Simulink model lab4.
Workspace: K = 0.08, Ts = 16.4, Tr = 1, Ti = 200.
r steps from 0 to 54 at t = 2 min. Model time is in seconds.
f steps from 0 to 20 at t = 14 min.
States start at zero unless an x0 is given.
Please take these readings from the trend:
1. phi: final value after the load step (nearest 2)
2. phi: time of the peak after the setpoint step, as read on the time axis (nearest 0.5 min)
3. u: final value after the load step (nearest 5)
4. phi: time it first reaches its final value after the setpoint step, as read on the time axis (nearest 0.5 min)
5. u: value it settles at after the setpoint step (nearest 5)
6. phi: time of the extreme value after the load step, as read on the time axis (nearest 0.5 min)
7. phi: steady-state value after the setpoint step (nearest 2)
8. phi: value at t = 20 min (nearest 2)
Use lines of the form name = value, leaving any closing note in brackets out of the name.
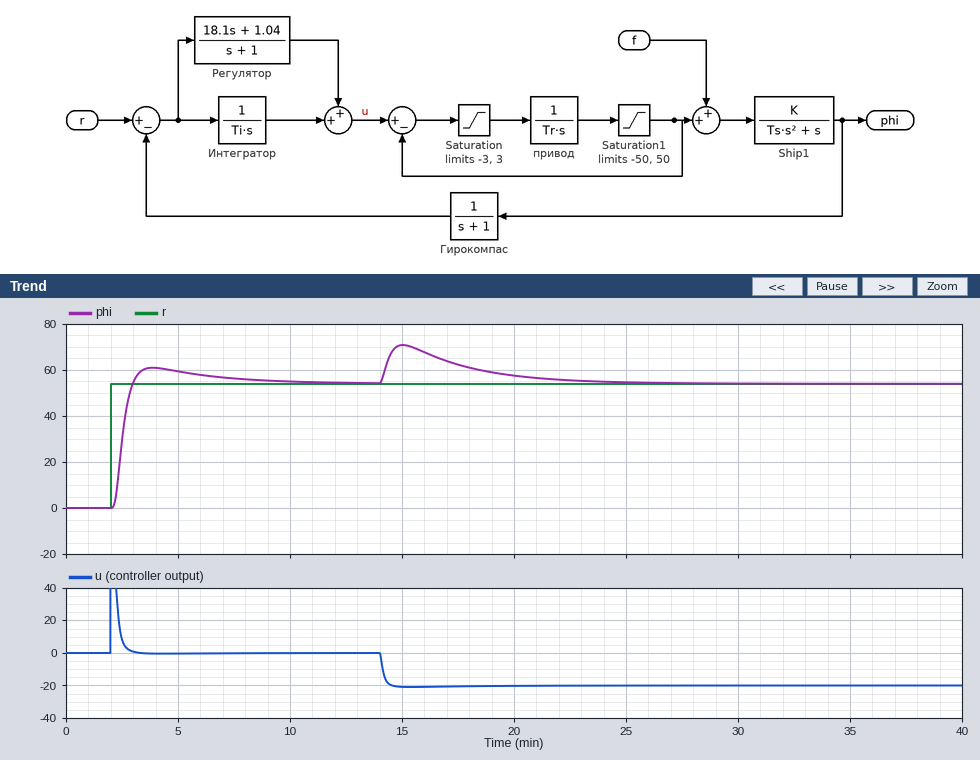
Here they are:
phi: final value after the load step = 54
phi: time of the peak after the setpoint step, as read on the time axis = 4.0 min
u: final value after the load step = -20
phi: time it first reaches its final value after the setpoint step, as read on the time axis = 3.0 min
u: value it settles at after the setpoint step = 0
phi: time of the extreme value after the load step, as read on the time axis = 15.0 min
phi: steady-state value after the setpoint step = 54
phi: value at t = 20 min = 58
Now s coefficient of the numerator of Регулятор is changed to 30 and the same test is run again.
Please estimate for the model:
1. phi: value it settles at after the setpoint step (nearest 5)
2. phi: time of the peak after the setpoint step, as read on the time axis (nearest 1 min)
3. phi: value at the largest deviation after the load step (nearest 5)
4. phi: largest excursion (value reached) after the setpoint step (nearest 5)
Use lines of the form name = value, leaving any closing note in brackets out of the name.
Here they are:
phi: value it settles at after the setpoint step = 55
phi: time of the peak after the setpoint step, as read on the time axis = 5 min
phi: value at the largest deviation after the load step = 70
phi: largest excursion (value reached) after the setpoint step = 60
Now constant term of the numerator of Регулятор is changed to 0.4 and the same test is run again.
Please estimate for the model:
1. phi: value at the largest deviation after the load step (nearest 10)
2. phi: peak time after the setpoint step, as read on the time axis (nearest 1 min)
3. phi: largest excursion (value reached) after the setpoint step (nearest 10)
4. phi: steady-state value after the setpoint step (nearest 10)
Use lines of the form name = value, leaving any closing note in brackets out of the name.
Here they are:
phi: value at the largest deviation after the load step = 80
phi: peak time after the setpoint step, as read on the time axis = 5 min
phi: largest excursion (value reached) after the setpoint step = 70
phi: steady-state value after the setpoint step = 50
